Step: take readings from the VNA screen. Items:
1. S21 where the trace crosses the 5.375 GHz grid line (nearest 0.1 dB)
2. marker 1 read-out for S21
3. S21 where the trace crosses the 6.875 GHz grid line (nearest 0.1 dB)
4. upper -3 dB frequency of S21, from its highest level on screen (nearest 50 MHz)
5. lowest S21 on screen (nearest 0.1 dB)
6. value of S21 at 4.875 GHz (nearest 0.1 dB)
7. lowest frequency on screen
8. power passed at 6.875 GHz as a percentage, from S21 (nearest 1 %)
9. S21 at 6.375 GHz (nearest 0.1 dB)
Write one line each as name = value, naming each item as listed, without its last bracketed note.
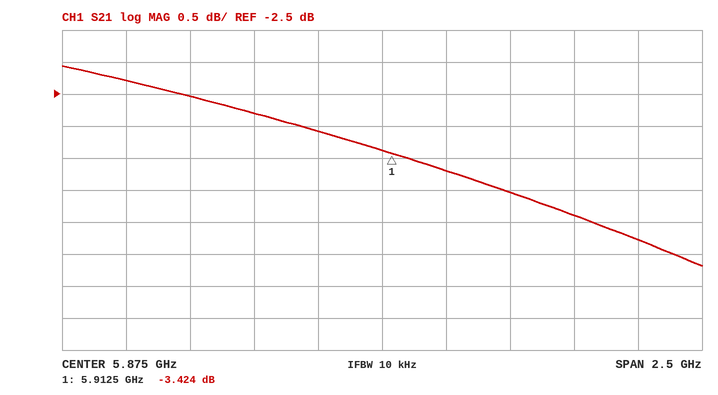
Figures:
S21 where the trace crosses the 5.375 GHz grid line = -2.8 dB
marker 1 read-out for S21 = -3.424 dB
S21 where the trace crosses the 6.875 GHz grid line = -4.8 dB
upper -3 dB frequency of S21, from its highest level on screen = 7.05 GHz
lowest S21 on screen = -5.2 dB
value of S21 at 4.875 GHz = -2.3 dB
lowest frequency on screen = 4.625 GHz
power passed at 6.875 GHz as a percentage, from S21 = 33 %
S21 at 6.375 GHz = -4.0 dB
